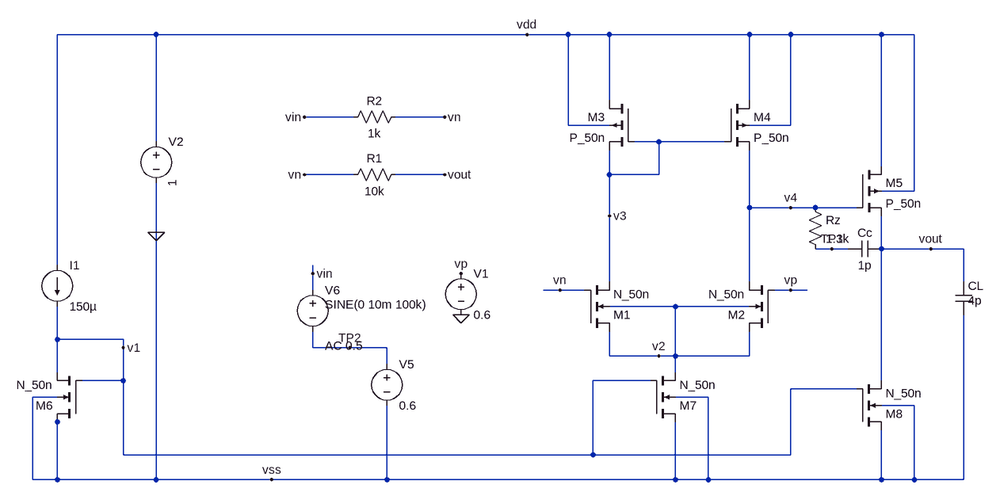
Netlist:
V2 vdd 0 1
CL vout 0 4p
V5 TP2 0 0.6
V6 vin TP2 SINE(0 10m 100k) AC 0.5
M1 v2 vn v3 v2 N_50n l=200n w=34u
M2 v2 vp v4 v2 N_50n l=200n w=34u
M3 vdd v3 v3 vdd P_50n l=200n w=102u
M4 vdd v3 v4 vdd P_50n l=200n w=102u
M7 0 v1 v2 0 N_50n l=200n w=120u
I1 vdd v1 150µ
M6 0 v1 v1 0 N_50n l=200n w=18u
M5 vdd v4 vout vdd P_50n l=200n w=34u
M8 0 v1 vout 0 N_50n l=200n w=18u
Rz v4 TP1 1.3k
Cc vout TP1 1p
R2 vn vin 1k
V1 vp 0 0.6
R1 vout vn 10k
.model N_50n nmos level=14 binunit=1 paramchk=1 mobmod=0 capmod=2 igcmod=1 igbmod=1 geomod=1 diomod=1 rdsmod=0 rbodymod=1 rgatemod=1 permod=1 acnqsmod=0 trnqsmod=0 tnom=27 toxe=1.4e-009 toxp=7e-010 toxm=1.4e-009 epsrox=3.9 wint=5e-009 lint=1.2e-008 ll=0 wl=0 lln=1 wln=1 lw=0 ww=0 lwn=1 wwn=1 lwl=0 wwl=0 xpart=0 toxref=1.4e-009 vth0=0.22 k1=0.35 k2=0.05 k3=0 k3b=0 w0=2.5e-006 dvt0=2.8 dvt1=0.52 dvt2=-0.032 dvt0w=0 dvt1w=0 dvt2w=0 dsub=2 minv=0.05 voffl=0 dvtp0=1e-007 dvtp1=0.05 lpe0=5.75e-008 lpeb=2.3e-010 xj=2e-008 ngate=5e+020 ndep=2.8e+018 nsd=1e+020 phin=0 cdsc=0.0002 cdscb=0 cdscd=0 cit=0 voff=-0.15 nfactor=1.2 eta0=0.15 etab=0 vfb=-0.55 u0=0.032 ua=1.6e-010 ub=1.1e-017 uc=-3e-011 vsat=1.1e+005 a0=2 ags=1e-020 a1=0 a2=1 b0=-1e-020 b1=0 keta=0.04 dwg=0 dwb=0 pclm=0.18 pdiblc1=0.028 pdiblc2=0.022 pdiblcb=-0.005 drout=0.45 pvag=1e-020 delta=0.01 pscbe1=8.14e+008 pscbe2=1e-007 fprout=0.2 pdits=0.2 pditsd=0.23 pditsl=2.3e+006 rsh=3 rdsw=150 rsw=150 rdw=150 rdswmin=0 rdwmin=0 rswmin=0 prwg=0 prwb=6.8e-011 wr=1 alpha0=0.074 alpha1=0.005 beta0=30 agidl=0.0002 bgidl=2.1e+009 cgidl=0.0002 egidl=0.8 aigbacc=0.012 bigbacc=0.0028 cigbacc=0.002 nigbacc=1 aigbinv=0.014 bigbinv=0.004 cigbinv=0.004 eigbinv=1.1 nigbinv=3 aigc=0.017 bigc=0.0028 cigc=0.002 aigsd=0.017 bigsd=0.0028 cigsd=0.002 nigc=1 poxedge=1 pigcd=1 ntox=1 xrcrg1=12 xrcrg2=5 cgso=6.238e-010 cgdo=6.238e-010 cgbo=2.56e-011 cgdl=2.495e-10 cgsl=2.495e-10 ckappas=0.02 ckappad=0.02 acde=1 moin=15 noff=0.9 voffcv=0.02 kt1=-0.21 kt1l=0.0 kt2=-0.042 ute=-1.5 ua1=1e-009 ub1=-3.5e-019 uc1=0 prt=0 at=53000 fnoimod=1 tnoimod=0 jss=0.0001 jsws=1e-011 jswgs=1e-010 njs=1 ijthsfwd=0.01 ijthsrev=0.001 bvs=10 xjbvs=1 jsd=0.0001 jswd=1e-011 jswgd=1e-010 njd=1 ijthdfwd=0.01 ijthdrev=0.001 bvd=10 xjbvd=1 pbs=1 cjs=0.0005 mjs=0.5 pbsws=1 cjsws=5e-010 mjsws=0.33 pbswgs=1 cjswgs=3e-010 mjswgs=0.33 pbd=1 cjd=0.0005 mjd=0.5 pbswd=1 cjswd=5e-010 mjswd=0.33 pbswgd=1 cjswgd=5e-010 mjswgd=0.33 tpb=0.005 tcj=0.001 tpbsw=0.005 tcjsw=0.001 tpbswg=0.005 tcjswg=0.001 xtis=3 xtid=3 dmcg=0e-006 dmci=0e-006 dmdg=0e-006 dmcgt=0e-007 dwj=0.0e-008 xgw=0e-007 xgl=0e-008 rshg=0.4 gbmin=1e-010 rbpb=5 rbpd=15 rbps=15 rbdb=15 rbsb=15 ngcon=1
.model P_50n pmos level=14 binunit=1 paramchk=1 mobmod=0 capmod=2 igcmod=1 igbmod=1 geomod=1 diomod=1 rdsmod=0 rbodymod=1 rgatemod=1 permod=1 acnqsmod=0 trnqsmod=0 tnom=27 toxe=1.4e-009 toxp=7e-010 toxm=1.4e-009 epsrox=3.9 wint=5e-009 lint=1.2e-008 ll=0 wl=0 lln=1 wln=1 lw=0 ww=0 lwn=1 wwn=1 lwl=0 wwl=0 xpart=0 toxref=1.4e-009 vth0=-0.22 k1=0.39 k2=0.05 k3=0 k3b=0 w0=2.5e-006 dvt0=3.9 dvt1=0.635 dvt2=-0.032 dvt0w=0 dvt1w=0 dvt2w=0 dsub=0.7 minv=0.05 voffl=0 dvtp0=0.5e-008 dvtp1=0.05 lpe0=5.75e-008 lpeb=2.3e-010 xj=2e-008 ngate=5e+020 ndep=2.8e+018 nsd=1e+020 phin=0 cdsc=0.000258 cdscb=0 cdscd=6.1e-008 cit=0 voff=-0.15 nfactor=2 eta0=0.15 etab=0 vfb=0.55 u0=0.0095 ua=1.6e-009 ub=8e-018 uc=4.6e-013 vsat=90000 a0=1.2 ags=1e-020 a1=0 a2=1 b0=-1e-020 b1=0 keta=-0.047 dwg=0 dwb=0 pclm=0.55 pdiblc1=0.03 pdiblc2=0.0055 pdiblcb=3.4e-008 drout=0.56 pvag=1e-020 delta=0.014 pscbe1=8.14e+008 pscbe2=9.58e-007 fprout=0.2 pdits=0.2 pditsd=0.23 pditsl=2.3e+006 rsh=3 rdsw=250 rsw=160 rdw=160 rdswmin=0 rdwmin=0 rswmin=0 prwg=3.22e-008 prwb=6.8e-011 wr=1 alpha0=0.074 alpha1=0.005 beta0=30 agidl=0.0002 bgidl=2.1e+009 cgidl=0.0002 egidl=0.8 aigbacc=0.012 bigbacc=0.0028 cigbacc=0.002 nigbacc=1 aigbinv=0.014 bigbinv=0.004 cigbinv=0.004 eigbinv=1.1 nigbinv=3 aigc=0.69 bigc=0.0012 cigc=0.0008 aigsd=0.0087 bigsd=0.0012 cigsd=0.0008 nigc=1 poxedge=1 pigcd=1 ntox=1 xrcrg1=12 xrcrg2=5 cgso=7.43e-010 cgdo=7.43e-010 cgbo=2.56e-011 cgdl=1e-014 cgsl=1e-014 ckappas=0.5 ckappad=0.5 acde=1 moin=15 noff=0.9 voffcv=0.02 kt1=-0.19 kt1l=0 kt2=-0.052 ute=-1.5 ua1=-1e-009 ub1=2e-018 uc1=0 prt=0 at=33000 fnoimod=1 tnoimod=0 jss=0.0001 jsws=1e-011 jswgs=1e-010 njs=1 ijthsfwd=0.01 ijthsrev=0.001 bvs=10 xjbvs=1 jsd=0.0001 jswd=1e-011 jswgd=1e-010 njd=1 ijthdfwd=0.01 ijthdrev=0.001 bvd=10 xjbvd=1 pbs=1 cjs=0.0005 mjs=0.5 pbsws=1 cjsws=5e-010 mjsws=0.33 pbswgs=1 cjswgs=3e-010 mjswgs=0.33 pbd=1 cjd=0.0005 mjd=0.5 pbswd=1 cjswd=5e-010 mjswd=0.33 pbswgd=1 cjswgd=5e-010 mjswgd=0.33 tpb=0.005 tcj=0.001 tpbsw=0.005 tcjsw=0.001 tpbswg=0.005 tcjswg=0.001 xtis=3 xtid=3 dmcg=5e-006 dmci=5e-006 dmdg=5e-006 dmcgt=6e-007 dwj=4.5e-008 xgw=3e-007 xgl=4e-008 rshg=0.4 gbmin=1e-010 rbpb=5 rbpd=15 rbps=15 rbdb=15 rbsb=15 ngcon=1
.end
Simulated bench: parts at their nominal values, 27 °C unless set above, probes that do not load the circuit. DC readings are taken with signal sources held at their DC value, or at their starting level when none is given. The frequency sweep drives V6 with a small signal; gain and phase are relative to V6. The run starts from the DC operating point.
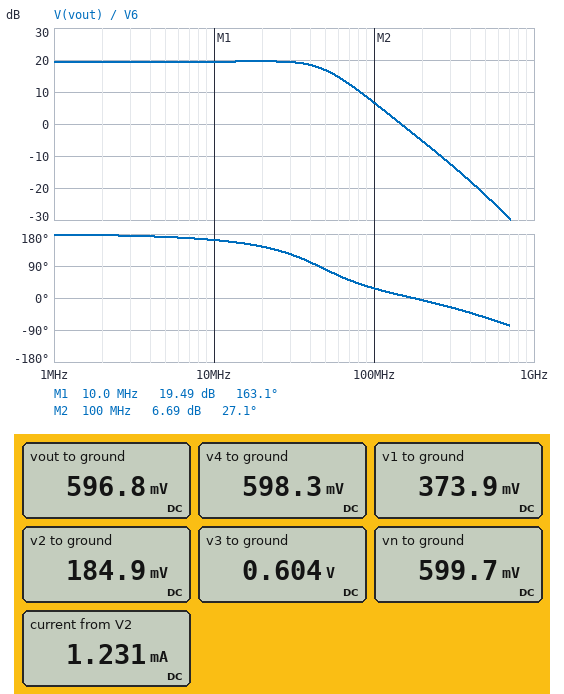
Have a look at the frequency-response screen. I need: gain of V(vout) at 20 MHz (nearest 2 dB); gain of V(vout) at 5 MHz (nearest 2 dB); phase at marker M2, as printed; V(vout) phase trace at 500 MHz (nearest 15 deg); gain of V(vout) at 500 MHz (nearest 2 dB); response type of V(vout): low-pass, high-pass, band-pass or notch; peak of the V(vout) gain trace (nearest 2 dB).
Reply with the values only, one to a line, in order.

20 dB
20 dB
27.1 deg
-60 deg
-22 dB
low-pass
20 dB
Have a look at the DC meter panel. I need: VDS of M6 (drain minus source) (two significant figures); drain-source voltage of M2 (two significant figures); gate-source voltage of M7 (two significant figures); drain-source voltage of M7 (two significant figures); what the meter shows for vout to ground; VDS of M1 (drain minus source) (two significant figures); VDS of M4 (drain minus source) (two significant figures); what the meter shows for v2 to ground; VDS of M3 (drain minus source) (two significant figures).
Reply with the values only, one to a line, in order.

-370 mV
-410 mV
190 mV
-180 mV
596.8 mV
-420 mV
400 mV
184.9 mV
400 mV
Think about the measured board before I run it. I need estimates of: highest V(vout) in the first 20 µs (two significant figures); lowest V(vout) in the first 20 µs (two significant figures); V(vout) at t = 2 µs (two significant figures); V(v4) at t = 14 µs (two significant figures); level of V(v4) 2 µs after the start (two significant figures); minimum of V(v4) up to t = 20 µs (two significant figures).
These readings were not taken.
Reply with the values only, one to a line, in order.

690 mV
500 mV
510 mV
600 mV
610 mV
590 mV
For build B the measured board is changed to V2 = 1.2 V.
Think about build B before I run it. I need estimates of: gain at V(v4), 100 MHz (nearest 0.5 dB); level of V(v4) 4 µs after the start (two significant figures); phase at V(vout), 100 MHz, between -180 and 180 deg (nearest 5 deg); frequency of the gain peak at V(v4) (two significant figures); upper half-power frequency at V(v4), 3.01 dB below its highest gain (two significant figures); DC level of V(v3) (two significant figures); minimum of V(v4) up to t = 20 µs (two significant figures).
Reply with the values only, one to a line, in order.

13.5 dB
810 mV
30 deg
49 MHz
92 MHz
800 mV
790 mV
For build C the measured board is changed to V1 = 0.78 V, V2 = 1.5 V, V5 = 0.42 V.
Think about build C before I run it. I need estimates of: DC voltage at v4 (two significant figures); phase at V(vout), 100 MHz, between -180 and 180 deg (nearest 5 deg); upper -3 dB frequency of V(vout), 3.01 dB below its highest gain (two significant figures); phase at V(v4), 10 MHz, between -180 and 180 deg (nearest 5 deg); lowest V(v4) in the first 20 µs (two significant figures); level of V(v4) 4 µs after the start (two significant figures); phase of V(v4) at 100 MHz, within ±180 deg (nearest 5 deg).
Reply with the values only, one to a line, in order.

170 mV
5 deg
380 MHz
0 deg
160 mV
180 mV
-15 deg
